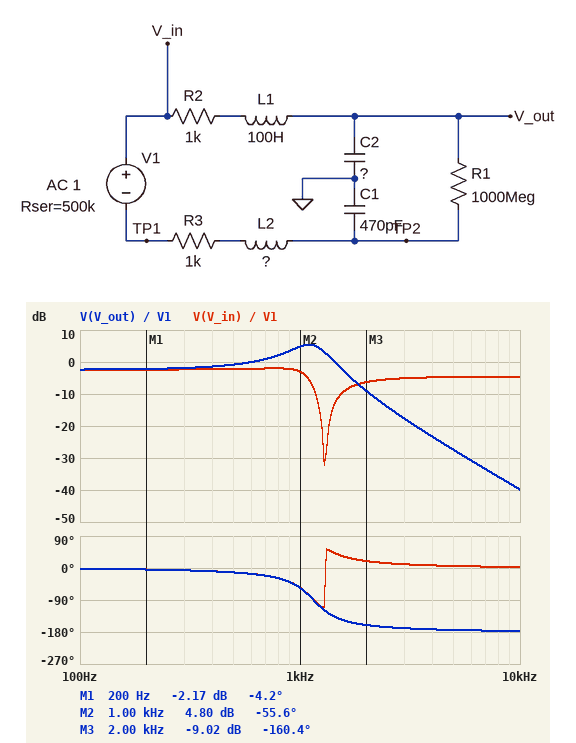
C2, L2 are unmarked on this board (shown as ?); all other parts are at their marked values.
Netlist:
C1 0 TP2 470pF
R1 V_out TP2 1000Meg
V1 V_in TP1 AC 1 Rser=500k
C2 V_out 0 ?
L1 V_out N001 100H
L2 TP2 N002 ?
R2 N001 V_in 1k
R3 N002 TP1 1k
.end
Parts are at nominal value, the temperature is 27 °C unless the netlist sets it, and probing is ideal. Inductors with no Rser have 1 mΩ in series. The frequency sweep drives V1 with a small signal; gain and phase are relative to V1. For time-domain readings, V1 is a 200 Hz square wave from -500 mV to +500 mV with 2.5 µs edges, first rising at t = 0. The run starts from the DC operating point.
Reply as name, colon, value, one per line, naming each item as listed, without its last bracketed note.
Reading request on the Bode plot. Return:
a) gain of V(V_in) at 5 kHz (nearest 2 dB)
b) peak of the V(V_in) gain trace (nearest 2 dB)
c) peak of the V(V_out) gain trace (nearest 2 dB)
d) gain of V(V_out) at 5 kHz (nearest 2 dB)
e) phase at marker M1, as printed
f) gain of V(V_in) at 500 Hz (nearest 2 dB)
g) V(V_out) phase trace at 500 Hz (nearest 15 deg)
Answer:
gain of V(V_in) at 5 kHz: -4 dB
peak of the V(V_in) gain trace: -2 dB
peak of the V(V_out) gain trace: 6 dB
gain of V(V_out) at 5 kHz: -28 dB
phase at marker M1, as printed: -4.2 deg
gain of V(V_in) at 500 Hz: -2 dB
V(V_out) phase trace at 500 Hz: -15 deg
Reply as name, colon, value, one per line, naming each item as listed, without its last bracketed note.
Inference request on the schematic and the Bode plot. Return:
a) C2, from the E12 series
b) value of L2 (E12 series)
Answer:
C2, from the E12 series: 150 pF
value of L2: 68 H
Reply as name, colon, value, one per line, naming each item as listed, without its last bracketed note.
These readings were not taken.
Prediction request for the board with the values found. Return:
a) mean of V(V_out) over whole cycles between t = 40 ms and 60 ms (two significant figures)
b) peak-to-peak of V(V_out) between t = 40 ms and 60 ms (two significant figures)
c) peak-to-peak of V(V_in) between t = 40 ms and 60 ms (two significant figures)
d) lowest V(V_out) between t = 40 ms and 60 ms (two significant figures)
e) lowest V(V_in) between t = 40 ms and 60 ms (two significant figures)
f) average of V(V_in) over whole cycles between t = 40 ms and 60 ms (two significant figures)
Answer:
mean of V(V_out) over whole cycles between t = 40 ms and 60 ms: 130 mV
peak-to-peak of V(V_out) between t = 40 ms and 60 ms: 1.5 V
peak-to-peak of V(V_in) between t = 40 ms and 60 ms: 1.0 V
lowest V(V_out) between t = 40 ms and 60 ms: -640 mV
lowest V(V_in) between t = 40 ms and 60 ms: -390 mV
average of V(V_in) over whole cycles between t = 40 ms and 60 ms: 130 mV
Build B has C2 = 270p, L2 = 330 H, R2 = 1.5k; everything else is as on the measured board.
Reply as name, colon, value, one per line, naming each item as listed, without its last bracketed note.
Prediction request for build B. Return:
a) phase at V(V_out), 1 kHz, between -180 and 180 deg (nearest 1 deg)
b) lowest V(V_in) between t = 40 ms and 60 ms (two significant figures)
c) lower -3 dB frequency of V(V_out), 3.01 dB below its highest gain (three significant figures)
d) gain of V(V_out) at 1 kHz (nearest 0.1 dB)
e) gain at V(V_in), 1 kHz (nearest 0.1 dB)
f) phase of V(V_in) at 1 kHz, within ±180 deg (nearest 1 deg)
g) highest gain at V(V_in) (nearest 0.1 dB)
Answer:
phase at V(V_out), 1 kHz, between -180 and 180 deg: -164 deg
lowest V(V_in) between t = 40 ms and 60 ms: -560 mV
lower -3 dB frequency of V(V_out), 3.01 dB below its highest gain: 467 Hz
gain of V(V_out) at 1 kHz: -9.9 dB
gain at V(V_in), 1 kHz: -33.5 dB
phase of V(V_in) at 1 kHz, within ±180 deg: 13 deg
highest gain at V(V_in): 2.5 dB
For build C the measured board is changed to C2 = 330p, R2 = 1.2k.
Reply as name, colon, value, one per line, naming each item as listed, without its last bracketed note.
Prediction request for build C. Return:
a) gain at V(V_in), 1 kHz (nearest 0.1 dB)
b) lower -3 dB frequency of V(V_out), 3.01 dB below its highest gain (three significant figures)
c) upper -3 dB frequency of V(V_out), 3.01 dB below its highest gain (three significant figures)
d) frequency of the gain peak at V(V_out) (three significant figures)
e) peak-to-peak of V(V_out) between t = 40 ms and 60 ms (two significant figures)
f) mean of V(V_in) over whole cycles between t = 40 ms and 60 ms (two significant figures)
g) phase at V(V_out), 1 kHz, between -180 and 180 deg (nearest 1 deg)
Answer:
gain at V(V_in), 1 kHz: -11.6 dB
lower -3 dB frequency of V(V_out), 3.01 dB below its highest gain: 510 Hz
upper -3 dB frequency of V(V_out), 3.01 dB below its highest gain: 1.03 kHz
frequency of the gain peak at V(V_out): 815 Hz
peak-to-peak of V(V_out) between t = 40 ms and 60 ms: 1.1 V
mean of V(V_in) over whole cycles between t = 40 ms and 60 ms: 44 mV
phase at V(V_out), 1 kHz, between -180 and 180 deg: -115 deg
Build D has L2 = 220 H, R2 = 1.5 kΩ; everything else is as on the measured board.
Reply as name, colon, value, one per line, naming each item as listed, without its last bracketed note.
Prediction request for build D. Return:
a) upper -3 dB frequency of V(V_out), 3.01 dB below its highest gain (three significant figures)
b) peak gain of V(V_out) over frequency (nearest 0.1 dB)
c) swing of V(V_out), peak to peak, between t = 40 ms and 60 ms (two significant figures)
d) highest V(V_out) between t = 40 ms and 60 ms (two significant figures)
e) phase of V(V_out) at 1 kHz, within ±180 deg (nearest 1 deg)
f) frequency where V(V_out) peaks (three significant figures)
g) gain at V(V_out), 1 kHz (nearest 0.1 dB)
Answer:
upper -3 dB frequency of V(V_out), 3.01 dB below its highest gain: 934 Hz
peak gain of V(V_out) over frequency: 8.1 dB
swing of V(V_out), peak to peak, between t = 40 ms and 60 ms: 1.6 V
highest V(V_out) between t = 40 ms and 60 ms: 920 mV
phase of V(V_out) at 1 kHz, within ±180 deg: -140 deg
frequency where V(V_out) peaks: 815 Hz
gain at V(V_out), 1 kHz: 2.5 dB
